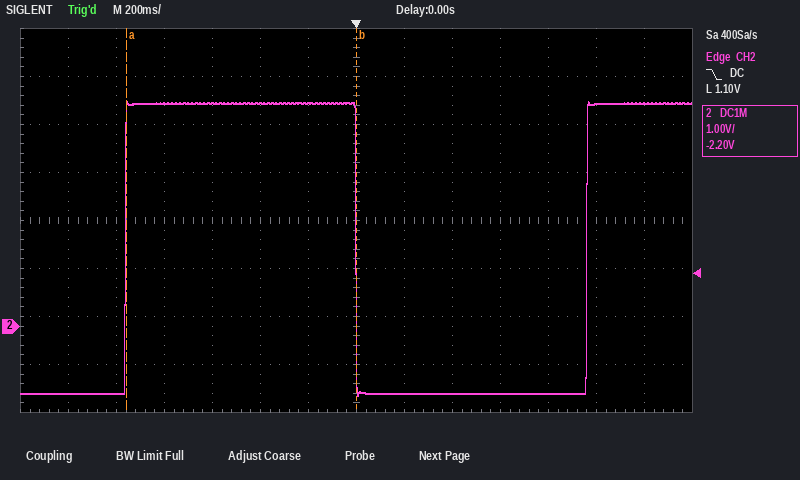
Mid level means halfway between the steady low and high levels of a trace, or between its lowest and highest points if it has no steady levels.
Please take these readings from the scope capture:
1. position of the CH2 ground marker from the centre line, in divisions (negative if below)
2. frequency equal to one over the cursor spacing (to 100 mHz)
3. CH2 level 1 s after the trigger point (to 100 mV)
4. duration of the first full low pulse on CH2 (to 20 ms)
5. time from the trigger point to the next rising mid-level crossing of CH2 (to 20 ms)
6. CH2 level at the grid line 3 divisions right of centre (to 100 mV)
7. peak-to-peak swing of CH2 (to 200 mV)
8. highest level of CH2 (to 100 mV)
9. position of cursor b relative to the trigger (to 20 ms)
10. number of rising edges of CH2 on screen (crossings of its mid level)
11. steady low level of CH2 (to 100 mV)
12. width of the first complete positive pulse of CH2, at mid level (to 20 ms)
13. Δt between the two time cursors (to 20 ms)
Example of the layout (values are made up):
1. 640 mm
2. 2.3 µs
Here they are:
1. -2.2 div
2. 1.0 Hz
3. 4.6 V
4. 960 ms
5. 960 ms
6. -1.4 V
7. 6.2 V
8. 4.7 V
9. 0 ms
10. 2
11. -1.4 V
12. 960 ms
13. 960 ms
